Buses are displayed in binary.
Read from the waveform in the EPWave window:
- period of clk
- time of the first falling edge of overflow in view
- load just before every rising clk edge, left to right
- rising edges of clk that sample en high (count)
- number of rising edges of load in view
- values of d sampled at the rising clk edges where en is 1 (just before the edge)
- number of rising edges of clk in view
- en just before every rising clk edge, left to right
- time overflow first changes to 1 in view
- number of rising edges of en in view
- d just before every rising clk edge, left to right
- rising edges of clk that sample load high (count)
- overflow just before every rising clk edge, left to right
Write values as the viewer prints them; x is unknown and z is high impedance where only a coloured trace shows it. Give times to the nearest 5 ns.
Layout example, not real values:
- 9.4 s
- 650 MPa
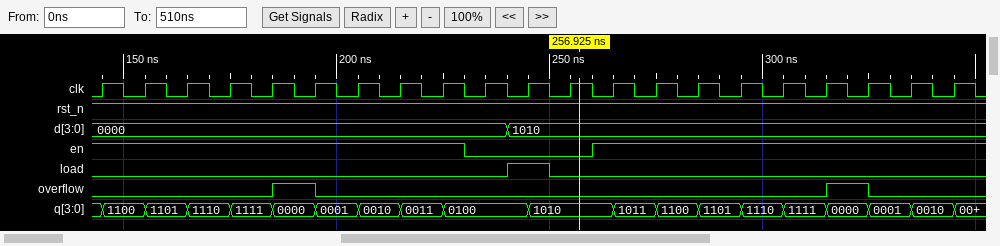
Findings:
- 10 ns
- 195 ns
- 0 0 0 0 0 0 0 0 0 0 1 0 0 0 0 0 0 0 0 0 0
- 18
- 1
- 0000, 0000, 0000, 0000, 0000, 0000, 0000, 0000, 0000, 1010, 1010, 1010, 1010, 1010, 1010, 1010, 1010, 1010
- 21
- 1 1 1 1 1 1 1 1 1 0 0 0 1 1 1 1 1 1 1 1 1
- 185 ns
- 1
- 0000, 0000, 0000, 0000, 0000, 0000, 0000, 0000, 0000, 0000, 1010, 1010, 1010, 1010, 1010, 1010, 1010, 1010, 1010, 1010, 1010
- 1
- 0 0 0 0 0 1 0 0 0 0 0 0 0 0 0 0 0 0 1 0 0
